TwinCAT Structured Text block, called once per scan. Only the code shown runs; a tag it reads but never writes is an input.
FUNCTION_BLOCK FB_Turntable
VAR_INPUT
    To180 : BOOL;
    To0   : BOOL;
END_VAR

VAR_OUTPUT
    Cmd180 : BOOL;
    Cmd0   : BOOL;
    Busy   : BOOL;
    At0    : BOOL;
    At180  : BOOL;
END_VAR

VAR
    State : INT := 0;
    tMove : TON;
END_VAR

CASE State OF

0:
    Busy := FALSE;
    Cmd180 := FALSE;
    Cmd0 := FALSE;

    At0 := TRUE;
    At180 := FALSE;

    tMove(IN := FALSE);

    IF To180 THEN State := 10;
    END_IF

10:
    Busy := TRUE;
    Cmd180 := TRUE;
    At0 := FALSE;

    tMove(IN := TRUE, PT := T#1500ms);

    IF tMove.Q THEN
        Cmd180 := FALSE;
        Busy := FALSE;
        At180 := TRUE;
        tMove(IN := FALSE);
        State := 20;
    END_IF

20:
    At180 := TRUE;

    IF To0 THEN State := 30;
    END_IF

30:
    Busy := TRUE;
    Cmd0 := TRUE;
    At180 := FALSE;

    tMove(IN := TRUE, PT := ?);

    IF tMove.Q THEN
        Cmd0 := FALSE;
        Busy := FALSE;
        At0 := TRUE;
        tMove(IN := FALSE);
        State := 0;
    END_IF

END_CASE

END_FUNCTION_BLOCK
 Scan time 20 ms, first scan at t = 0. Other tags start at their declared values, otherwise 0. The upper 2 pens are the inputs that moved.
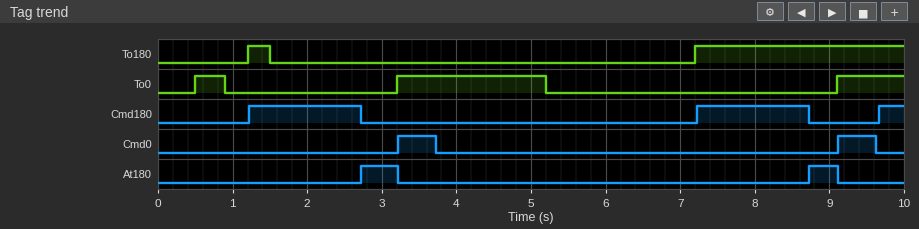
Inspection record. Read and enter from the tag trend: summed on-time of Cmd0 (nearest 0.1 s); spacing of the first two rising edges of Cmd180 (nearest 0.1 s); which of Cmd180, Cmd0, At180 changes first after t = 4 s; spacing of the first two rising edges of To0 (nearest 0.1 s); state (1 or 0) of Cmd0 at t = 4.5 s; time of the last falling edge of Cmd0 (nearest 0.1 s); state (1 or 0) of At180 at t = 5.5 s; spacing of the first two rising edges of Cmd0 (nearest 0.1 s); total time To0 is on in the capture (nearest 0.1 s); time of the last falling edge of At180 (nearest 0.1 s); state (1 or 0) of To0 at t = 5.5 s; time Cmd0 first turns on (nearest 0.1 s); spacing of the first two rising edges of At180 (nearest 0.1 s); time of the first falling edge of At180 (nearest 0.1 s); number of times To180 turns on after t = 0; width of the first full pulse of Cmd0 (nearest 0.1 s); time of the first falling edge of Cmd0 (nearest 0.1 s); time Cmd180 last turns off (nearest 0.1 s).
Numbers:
1.0 s
6.0 s
Cmd180
2.7 s
0
9.6 s
0
5.9 s
3.3 s
9.1 s
0
3.2 s
6.0 s
3.2 s
2
0.5 s
3.7 s
8.7 s
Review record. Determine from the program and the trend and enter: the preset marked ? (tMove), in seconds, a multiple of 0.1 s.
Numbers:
0.5 s
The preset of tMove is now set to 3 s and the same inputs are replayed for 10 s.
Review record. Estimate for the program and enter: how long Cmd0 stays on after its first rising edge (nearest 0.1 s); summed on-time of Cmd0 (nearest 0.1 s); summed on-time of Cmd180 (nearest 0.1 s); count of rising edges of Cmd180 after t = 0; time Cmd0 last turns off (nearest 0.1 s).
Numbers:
3.0 s
3.9 s
3.0 s
2
6.2 s
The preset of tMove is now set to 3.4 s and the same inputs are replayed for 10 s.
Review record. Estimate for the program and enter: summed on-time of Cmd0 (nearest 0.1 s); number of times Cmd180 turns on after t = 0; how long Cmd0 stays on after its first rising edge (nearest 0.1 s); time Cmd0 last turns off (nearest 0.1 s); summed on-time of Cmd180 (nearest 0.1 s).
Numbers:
4.3 s
2
3.4 s
6.6 s
3.0 s
